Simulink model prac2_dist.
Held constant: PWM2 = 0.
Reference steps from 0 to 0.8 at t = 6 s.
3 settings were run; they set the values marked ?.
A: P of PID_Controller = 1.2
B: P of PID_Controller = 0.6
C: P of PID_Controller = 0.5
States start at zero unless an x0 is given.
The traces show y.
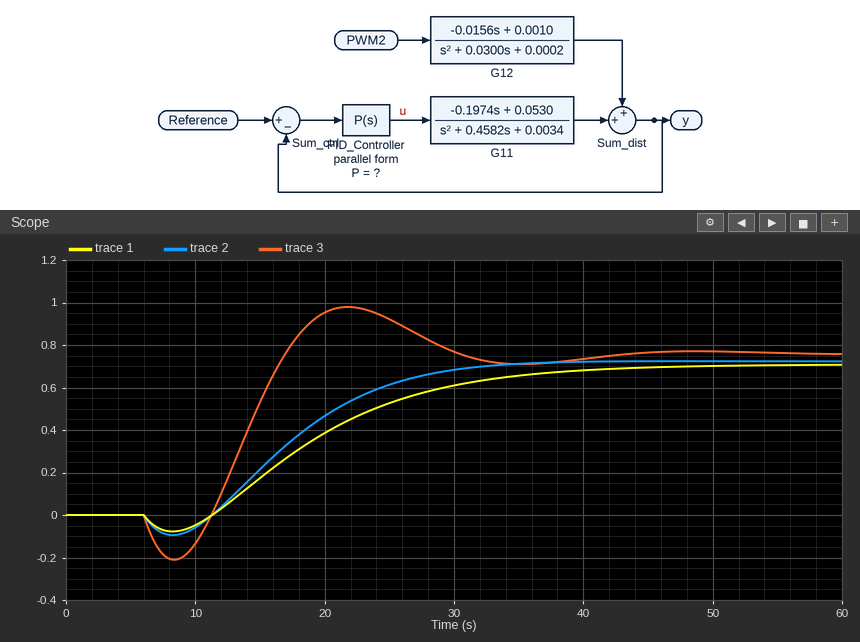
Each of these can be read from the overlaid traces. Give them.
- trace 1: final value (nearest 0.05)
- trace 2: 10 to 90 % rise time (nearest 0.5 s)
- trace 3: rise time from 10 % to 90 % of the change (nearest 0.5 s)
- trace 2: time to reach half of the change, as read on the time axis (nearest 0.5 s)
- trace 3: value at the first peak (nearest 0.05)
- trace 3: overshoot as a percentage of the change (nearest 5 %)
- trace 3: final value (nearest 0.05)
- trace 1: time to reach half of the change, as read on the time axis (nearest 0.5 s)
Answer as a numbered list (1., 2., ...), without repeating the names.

1. 0.70
2. 14.5 s
3. 4.5 s
4. 17.5 s
5. 1.00
6. 30 %
7. 0.75
8. 19.0 s
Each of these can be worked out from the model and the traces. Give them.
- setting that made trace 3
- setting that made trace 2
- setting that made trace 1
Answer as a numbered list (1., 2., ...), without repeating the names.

1. A
2. B
3. C
